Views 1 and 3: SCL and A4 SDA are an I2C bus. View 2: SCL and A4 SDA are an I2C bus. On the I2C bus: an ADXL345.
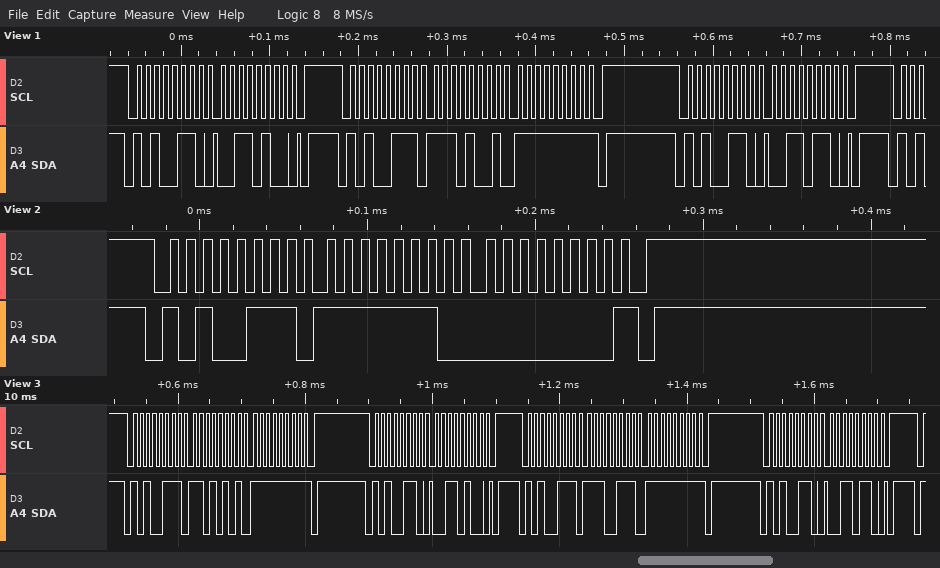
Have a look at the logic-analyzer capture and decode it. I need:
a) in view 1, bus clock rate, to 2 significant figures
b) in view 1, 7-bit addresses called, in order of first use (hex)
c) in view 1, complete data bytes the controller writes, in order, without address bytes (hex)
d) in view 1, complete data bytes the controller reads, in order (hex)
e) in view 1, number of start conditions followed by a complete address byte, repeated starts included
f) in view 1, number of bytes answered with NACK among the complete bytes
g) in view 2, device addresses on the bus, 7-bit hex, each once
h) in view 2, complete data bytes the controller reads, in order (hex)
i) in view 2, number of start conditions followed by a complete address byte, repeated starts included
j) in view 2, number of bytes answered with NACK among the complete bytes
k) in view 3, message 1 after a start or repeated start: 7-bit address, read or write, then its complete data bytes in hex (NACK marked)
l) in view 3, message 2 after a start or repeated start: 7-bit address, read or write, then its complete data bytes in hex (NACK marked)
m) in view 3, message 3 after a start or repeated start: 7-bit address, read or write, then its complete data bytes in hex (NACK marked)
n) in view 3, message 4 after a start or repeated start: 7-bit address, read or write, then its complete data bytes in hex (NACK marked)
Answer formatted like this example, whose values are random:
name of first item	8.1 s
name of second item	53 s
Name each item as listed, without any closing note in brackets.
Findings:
in view 1, bus clock rate, to 2 significant figures	100 kHz
in view 1, 7-bit addresses called, in order of first use	0x53
in view 1, complete data bytes the controller writes, in order, without address bytes	34 36
in view 1, complete data bytes the controller reads, in order	E9 FF
in view 1, number of start conditions followed by a complete address byte, repeated starts included	3
in view 1, number of bytes answered with NACK among the complete bytes	1
in view 2, device addresses on the bus, 7-bit hex, each once	0x53
in view 2, complete data bytes the controller reads, in order	FE 00
in view 2, number of start conditions followed by a complete address byte, repeated starts included	1
in view 2, number of bytes answered with NACK among the complete bytes	1
in view 3, message 1 after a start or repeated start: 7-bit address, read or write, then its complete data bytes in hex	0x53 read: D5 FF NACK
in view 3, message 2 after a start or repeated start: 7-bit address, read or write, then its complete data bytes in hex	0x53 write: 34
in view 3, message 3 after a start or repeated start: 7-bit address, read or write, then its complete data bytes in hex	0x53 read: E7 FF NACK
in view 3, message 4 after a start or repeated start: 7-bit address, read or write, then its complete data bytes in hex	0x53 write: 36
